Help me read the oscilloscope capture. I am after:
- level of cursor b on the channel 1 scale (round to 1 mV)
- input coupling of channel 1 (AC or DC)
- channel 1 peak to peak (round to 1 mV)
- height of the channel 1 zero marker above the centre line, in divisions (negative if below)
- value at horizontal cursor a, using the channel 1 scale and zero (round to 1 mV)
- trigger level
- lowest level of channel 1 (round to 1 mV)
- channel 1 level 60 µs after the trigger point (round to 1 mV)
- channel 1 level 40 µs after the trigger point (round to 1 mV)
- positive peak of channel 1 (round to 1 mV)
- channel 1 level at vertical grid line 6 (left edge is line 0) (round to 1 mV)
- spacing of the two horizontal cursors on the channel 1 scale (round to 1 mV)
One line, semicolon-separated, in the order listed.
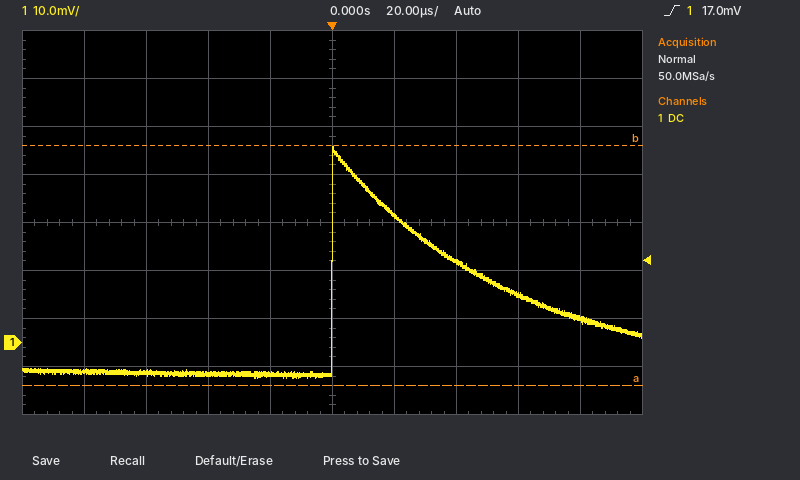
41 mV; DC; 48 mV; -2.5 div; -9 mV; 17.0 mV; -7 mV; 10 mV; 17 mV; 41 mV; 27 mV; 50 mV
